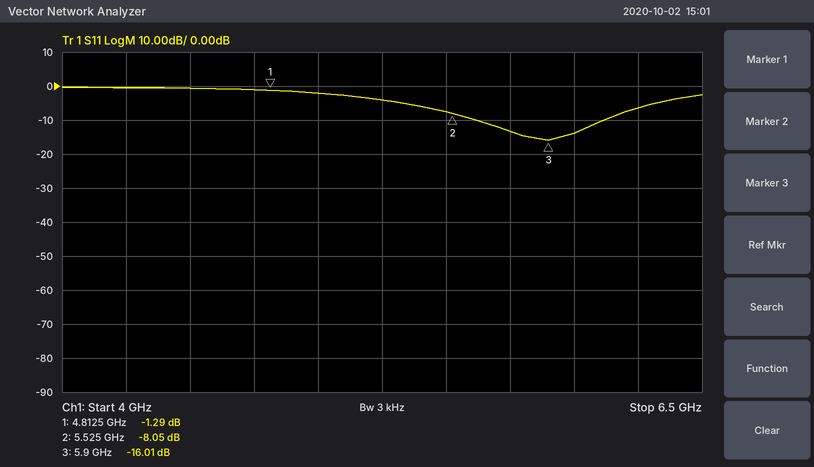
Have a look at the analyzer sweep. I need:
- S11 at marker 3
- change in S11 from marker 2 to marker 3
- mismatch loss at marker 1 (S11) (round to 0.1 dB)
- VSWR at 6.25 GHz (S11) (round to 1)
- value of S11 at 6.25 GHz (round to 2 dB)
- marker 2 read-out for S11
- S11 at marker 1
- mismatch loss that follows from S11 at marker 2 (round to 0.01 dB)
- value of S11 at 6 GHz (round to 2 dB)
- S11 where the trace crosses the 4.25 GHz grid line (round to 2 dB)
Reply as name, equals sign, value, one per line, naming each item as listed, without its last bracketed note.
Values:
S11 at marker 3 = -16.01 dB
change in S11 from marker 2 to marker 3 = -7.96 dB
mismatch loss at marker 1 (S11) = 5.9 dB
VSWR at 6.25 GHz (S11) = 3
value of S11 at 6.25 GHz = -6 dB
marker 2 read-out for S11 = -8.05 dB
S11 at marker 1 = -1.29 dB
mismatch loss that follows from S11 at marker 2 = 0.74 dB
value of S11 at 6 GHz = -14 dB
S11 where the trace crosses the 4.25 GHz grid line = 0 dB
